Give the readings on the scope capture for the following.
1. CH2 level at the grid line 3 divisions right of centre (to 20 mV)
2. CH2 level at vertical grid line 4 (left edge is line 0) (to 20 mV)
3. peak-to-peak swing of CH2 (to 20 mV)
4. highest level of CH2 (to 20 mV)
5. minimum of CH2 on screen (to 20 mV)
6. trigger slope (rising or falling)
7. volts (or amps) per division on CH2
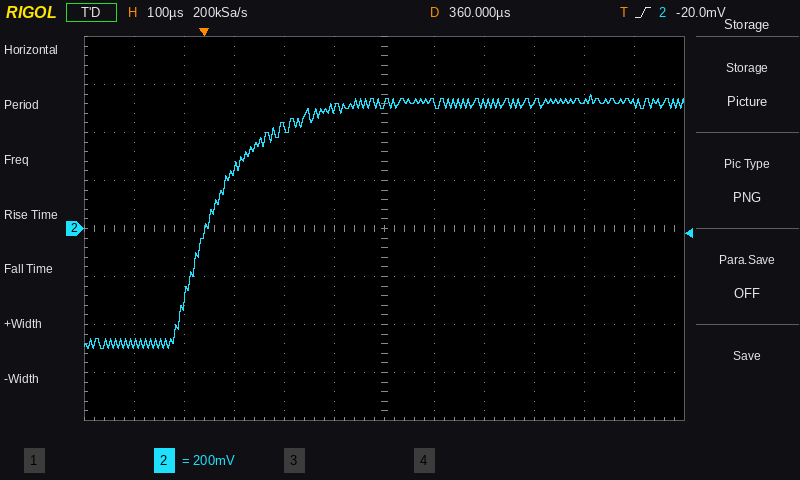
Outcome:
520 mV
420 mV
1.06 V
560 mV
-500 mV
rising
200 mV
